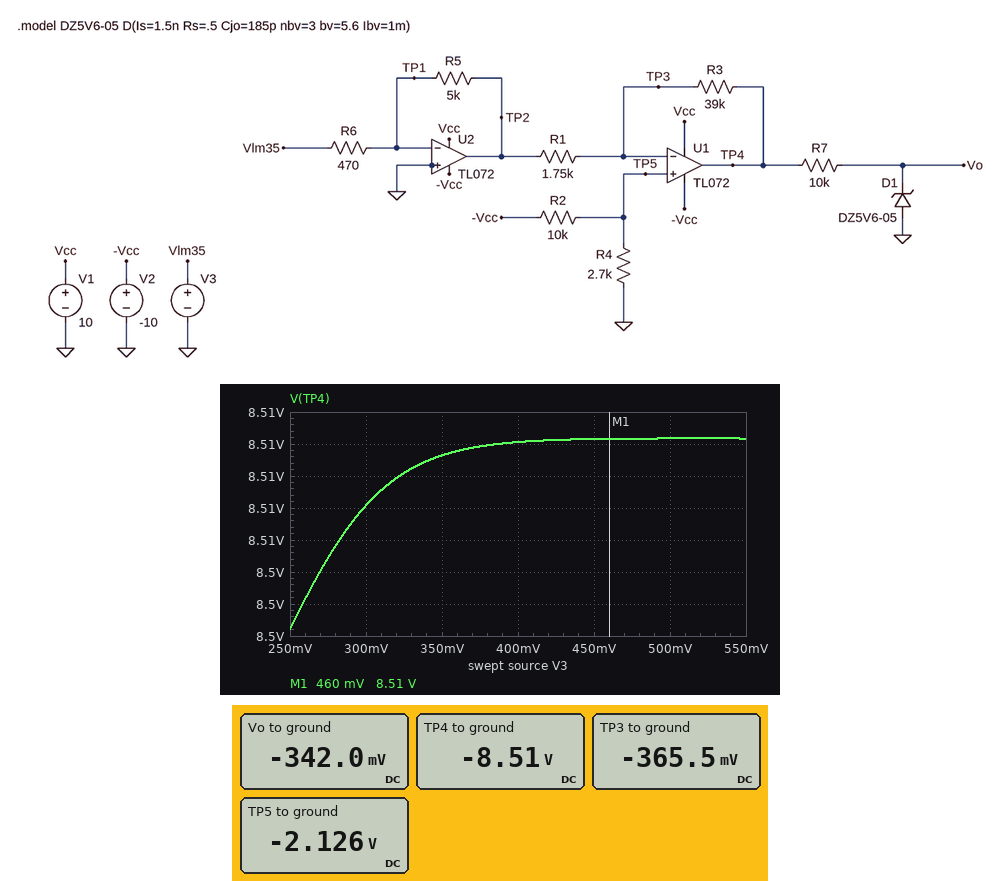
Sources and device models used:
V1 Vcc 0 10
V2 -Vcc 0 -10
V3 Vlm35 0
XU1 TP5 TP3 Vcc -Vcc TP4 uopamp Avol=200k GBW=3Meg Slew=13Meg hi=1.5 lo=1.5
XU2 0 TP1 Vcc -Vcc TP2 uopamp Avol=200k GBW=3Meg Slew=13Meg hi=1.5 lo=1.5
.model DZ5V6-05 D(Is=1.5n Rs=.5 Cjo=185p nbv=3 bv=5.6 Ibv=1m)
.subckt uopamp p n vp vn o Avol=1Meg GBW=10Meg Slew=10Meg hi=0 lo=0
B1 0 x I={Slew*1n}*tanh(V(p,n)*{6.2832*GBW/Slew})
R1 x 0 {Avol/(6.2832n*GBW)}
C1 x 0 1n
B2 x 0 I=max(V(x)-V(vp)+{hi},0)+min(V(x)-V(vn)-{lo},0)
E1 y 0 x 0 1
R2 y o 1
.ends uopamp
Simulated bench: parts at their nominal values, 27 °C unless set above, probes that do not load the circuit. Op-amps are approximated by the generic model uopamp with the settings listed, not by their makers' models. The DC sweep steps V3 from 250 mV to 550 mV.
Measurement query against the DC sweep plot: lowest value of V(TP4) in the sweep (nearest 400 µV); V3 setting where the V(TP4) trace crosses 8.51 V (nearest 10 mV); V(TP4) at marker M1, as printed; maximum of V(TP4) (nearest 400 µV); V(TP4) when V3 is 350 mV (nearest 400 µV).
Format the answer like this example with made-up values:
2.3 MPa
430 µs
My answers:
8.5004 V
320 mV
8.51 V
8.5124 V
8.5112 V
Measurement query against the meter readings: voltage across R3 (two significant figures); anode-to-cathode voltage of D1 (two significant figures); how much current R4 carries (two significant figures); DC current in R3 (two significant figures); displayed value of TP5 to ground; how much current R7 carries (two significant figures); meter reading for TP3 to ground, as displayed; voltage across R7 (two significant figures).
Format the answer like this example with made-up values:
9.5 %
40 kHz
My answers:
8.1 V
340 mV
790 µA
210 µA
-2.126 V
820 µA
-365.5 mV
8.2 V
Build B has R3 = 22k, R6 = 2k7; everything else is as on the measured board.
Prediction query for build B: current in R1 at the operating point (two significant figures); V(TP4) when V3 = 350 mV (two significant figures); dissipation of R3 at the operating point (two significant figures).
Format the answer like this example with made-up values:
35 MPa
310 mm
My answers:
360 µA
-8.5 V
2.8 mW
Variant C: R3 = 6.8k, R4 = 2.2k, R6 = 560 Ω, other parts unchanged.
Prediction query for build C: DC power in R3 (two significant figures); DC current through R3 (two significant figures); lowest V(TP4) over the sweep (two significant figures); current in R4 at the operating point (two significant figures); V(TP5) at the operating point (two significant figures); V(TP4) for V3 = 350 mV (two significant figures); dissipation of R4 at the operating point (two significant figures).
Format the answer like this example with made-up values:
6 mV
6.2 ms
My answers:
6.7 mW
990 µA
-140 mV
820 µA
-1.8 V
3.3 V
1.5 mW
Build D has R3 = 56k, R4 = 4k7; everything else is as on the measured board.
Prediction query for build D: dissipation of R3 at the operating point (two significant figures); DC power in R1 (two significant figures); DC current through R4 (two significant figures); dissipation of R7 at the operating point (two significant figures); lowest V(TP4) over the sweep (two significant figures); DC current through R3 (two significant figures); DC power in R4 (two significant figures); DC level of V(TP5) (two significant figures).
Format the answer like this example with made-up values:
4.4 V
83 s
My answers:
1.2 mW
38 µW
680 µA
6.7 mW
-8.5 V
150 µA
2.2 mW
-3.2 V
